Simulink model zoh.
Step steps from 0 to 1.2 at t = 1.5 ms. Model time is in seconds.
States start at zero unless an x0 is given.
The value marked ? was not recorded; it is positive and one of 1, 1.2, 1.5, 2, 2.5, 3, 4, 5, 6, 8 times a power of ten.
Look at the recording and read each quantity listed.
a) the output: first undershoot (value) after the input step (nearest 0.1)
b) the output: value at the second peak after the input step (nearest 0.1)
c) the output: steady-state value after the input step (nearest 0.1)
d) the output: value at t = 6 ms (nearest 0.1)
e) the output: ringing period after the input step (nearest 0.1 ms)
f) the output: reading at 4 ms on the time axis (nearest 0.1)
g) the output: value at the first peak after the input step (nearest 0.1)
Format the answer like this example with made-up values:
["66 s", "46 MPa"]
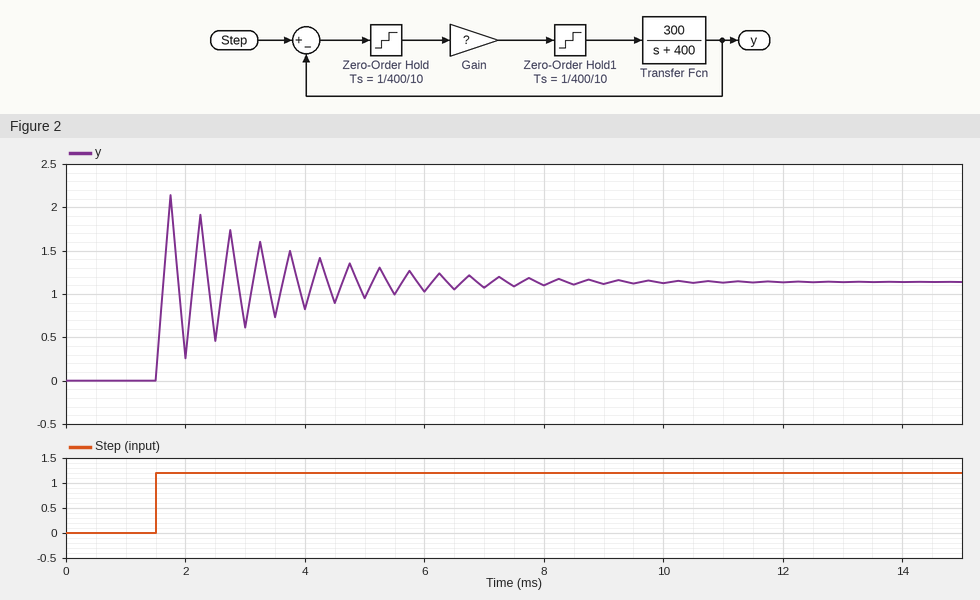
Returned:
["0.3", "1.9", "1.1", "1.0", "0.5 ms", "0.8", "2.1"]
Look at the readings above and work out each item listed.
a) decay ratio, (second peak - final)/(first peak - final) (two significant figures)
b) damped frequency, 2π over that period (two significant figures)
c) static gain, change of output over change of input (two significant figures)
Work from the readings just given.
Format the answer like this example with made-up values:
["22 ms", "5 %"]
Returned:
["0.80", "13 rad/ms", "0.92"]
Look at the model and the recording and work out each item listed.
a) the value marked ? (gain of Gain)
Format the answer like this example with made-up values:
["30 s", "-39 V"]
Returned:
["25"]
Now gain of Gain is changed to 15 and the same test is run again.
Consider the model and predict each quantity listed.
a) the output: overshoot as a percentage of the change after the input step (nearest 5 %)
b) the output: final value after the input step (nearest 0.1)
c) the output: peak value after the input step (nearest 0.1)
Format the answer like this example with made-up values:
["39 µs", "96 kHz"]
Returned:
["15 %", "1.1", "1.3"]
